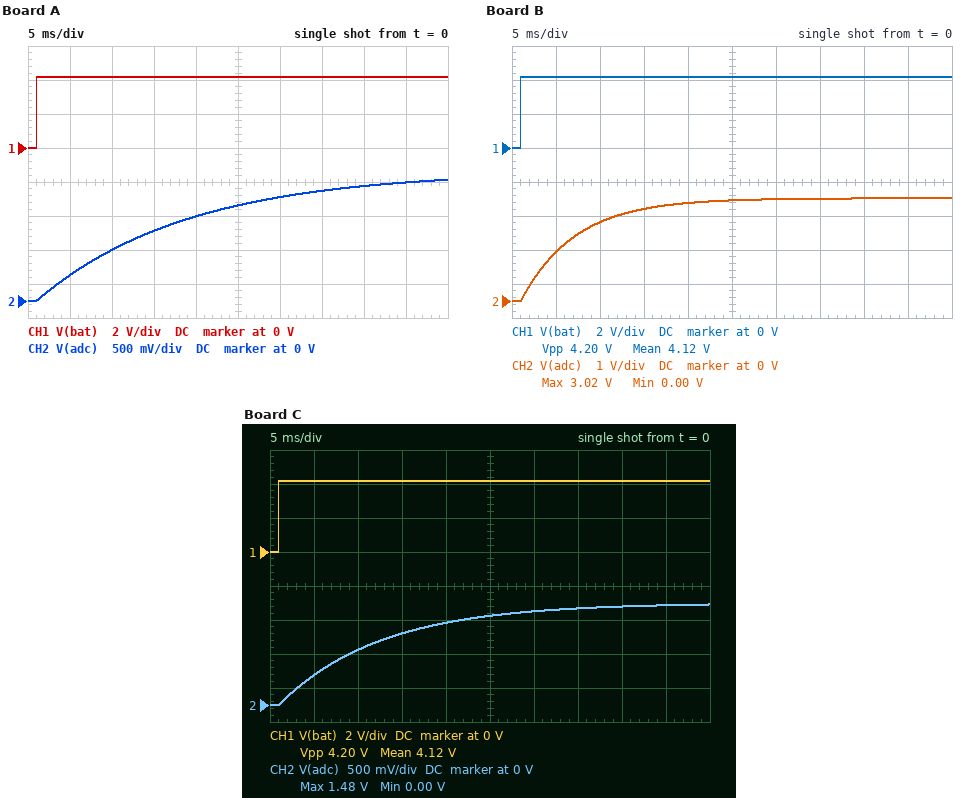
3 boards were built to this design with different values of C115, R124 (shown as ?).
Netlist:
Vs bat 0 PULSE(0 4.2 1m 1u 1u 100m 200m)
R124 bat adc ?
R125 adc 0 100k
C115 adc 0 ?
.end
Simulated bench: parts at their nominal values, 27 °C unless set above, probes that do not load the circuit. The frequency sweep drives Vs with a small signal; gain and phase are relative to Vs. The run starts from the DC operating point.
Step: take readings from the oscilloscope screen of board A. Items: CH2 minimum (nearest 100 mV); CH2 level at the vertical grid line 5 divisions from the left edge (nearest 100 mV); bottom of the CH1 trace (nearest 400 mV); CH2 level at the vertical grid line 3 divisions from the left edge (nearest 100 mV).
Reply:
0 V
1.4 V
0 V
1.0 V
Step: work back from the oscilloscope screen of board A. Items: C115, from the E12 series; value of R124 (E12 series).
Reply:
330 nF
120 kΩ
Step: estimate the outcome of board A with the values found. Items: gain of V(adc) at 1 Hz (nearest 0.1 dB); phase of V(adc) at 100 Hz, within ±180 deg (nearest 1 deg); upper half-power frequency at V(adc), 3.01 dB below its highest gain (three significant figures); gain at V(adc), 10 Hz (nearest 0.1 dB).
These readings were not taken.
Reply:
-6.9 dB
-85 deg
8.84 Hz
-10.4 dB
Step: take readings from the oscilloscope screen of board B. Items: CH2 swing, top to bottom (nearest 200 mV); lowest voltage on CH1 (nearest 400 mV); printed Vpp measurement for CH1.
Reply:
3.0 V
0 V
4.20 V
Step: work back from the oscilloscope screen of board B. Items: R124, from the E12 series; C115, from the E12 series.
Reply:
39 kΩ
220 nF
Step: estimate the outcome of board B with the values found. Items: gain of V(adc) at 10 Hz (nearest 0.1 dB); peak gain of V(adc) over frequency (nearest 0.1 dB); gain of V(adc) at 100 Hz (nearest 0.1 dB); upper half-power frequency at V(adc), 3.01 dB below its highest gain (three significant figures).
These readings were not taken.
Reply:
-3.5 dB
-2.9 dB
-14.9 dB
25.8 Hz
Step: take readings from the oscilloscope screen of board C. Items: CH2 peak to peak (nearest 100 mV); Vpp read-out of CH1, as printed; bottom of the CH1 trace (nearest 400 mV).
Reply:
1.5 V
4.20 V
0 V
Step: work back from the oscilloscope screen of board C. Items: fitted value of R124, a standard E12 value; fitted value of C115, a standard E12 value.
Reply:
180 kΩ
180 nF
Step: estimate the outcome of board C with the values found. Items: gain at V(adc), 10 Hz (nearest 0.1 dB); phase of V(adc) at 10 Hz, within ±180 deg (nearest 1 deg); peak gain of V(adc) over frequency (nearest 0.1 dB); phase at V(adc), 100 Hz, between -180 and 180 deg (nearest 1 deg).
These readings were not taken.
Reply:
-10.8 dB
-36 deg
-8.9 dB
-82 deg
